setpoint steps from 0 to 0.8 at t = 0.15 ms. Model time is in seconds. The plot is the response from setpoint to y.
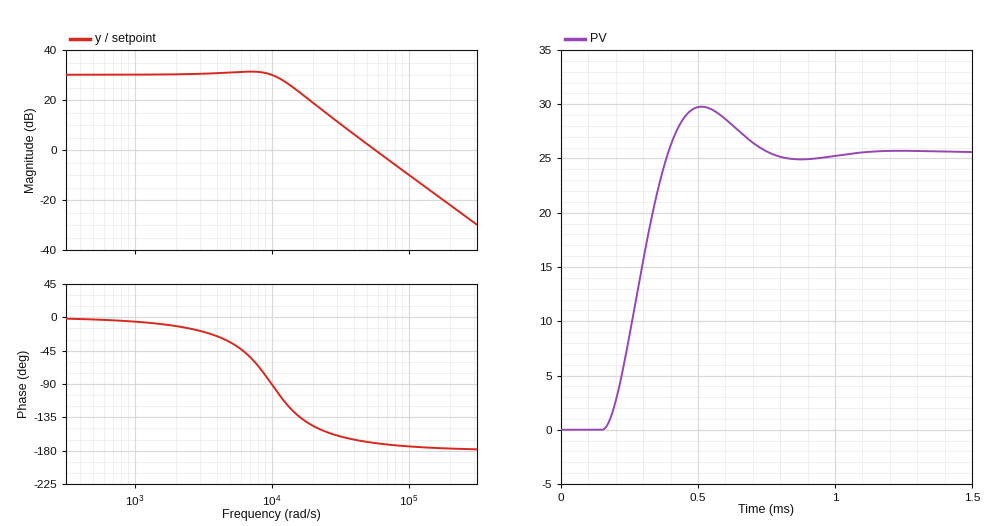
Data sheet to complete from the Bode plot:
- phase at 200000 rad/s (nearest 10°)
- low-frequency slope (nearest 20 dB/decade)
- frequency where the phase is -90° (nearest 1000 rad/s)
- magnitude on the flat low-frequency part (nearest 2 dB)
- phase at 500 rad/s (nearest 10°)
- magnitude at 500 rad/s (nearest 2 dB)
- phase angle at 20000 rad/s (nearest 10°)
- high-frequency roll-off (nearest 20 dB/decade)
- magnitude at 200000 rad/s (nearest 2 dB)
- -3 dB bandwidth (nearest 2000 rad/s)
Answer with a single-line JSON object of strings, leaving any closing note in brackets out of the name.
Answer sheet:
{"phase at 200000 rad/s": "-180°", "low-frequency slope": "0 dB/decade", "frequency where the phase is -90°": "10000 rad/s", "magnitude on the flat low-frequency part": "30 dB", "phase at 500 rad/s": "0°", "magnitude at 500 rad/s": "30 dB", "phase angle at 20000 rad/s": "-150°", "high-frequency roll-off": "-40 dB/decade", "magnitude at 200000 rad/s": "-22 dB", "-3 dB bandwidth": "12000 rad/s"}
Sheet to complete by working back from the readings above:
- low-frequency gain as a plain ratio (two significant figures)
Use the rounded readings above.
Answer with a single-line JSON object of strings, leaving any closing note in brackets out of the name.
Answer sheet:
{"low-frequency gain as a plain ratio": "32"}
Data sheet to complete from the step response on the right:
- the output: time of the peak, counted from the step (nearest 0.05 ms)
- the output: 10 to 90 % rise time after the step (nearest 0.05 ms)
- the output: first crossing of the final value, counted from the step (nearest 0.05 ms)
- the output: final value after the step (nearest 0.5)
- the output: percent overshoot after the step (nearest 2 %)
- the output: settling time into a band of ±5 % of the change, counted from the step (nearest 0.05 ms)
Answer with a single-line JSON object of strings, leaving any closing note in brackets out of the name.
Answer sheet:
{"the output: time of the peak, counted from the step": "0.35 ms", "the output: 10 to 90 % rise time after the step": "0.15 ms", "the output: first crossing of the final value, counted from the step": "0.25 ms", "the output: final value after the step": "25.5", "the output: percent overshoot after the step": "16 %", "the output: settling time into a band of ±5 % of the change, counted from the step": "0.55 ms"}
